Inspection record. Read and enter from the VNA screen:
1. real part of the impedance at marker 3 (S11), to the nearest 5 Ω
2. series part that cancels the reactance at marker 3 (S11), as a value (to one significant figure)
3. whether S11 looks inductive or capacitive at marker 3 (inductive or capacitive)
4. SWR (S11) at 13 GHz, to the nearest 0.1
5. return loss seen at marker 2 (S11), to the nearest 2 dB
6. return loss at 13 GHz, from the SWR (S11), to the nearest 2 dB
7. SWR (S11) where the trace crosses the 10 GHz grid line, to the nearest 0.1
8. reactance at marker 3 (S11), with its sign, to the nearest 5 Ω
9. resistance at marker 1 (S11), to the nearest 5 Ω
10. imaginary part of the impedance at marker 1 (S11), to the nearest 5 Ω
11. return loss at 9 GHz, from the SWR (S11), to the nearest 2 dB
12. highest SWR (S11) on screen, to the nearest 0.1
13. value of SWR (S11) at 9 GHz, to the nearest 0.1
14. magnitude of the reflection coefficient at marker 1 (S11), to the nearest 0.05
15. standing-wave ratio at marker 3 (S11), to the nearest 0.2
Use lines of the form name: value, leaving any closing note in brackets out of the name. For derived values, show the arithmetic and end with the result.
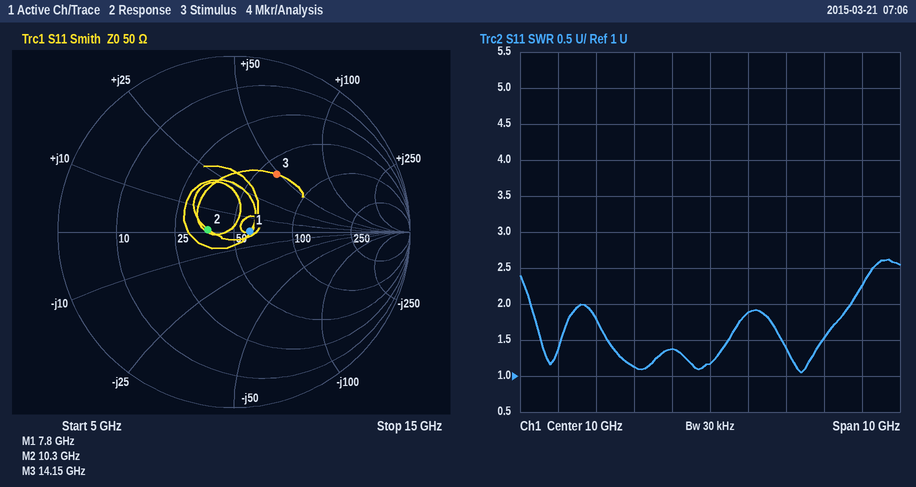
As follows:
real part of the impedance at marker 3 (S11), to the nearest 5 Ω: 60 Ω
series part that cancels the reactance at marker 3 (S11), as a value: C = 1/(2π × 14.15 GHz × 50 Ω) ≈ 225 fF, so 200 fF to one significant figure
whether S11 looks inductive or capacitive at marker 3: inductive
SWR (S11) at 13 GHz, to the nearest 0.1: 1.5
return loss seen at marker 2 (S11), to the nearest 2 dB: 16 dB
return loss at 13 GHz, from the SWR (S11), to the nearest 2 dB: −20 log10((1.5 − 1)/(1.5 + 1)) ≈ 14 dB
SWR (S11) where the trace crosses the 10 GHz grid line, to the nearest 0.1: 1.2
reactance at marker 3 (S11), with its sign, to the nearest 5 Ω: +50 Ω
resistance at marker 1 (S11), to the nearest 5 Ω: 60 Ω
imaginary part of the impedance at marker 1 (S11), to the nearest 5 Ω: 0 Ω
return loss at 9 GHz, from the SWR (S11), to the nearest 2 dB: −20 log10((1.4 − 1)/(1.4 + 1)) ≈ 16 dB
highest SWR (S11) on screen, to the nearest 0.1: 2.6
value of SWR (S11) at 9 GHz, to the nearest 0.1: 1.4
magnitude of the reflection coefficient at marker 1 (S11), to the nearest 0.05: 0.10
standing-wave ratio at marker 3 (S11), to the nearest 0.2: 2.4
